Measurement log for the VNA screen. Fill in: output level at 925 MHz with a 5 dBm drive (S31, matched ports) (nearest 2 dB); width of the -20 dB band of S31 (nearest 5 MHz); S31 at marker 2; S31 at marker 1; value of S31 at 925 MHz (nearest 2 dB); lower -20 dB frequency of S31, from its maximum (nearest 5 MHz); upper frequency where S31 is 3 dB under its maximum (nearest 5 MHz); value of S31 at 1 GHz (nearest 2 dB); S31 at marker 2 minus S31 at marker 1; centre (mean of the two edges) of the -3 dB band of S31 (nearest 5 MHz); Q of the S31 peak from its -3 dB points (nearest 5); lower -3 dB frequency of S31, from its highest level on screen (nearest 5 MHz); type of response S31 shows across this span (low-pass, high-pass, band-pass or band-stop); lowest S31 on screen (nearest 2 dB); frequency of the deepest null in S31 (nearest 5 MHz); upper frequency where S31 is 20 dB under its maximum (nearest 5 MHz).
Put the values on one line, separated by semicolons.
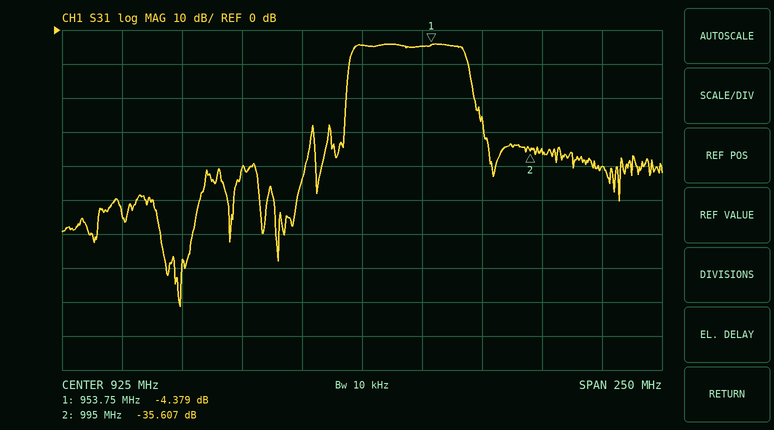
0 dBm; 55 MHz; -35.607 dB; -4.379 dB; -4 dB; 920 MHz; 970 MHz; -36 dB; -31.228 dB; 945 MHz; 20; 920 MHz; band-pass; -82 dB; 850 MHz; 975 MHz
